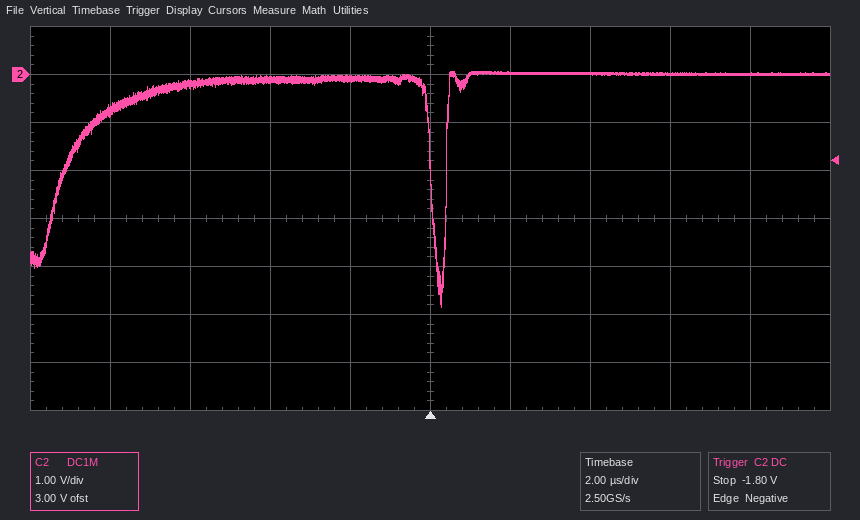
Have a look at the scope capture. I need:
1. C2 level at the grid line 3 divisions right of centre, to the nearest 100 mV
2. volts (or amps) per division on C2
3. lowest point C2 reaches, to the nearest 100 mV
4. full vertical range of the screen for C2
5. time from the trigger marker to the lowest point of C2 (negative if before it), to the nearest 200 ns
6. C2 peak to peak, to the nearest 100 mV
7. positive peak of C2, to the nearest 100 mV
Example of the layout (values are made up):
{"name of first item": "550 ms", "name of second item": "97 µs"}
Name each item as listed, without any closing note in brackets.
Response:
{"C2 level at the grid line 3 divisions right of centre, to the nearest 100 mV": "0.0 V", "volts (or amps) per division on C2": "1 V", "lowest point C2 reaches, to the nearest 100 mV": "-4.8 V", "full vertical range of the screen for C2": "8 V", "time from the trigger marker to the lowest point of C2 (negative if before it), to the nearest 200 ns": "+200 ns", "C2 peak to peak, to the nearest 100 mV": "4.9 V", "positive peak of C2, to the nearest 100 mV": "100 mV"}
